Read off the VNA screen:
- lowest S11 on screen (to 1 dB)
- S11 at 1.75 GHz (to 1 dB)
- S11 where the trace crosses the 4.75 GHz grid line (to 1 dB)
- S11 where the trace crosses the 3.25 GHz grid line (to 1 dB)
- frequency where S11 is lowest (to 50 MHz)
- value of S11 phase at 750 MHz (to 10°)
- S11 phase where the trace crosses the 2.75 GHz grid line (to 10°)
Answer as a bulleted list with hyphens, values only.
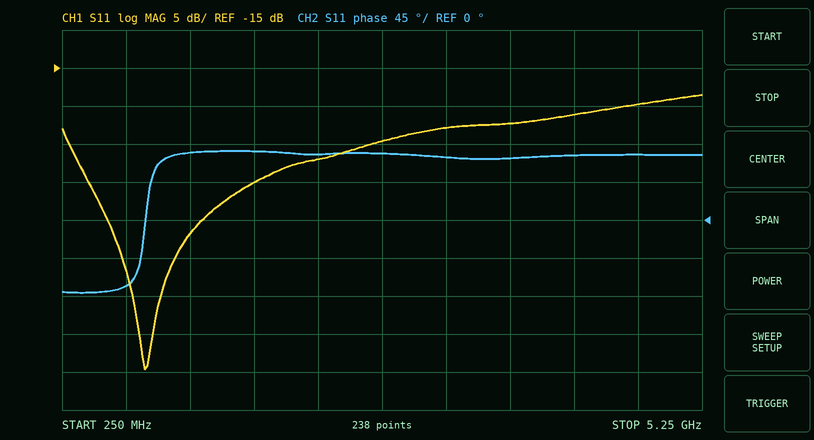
- -55 dB
- -30 dB
- -20 dB
- -23 dB
- 900 MHz
- -80°
- 80°
